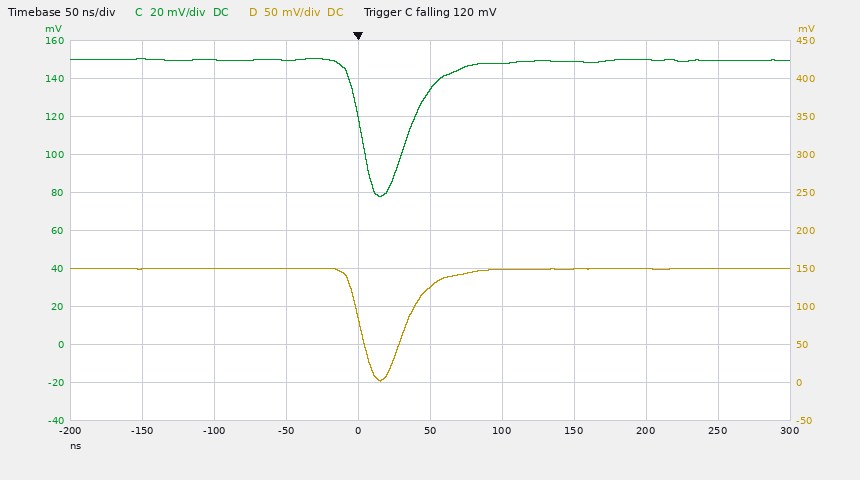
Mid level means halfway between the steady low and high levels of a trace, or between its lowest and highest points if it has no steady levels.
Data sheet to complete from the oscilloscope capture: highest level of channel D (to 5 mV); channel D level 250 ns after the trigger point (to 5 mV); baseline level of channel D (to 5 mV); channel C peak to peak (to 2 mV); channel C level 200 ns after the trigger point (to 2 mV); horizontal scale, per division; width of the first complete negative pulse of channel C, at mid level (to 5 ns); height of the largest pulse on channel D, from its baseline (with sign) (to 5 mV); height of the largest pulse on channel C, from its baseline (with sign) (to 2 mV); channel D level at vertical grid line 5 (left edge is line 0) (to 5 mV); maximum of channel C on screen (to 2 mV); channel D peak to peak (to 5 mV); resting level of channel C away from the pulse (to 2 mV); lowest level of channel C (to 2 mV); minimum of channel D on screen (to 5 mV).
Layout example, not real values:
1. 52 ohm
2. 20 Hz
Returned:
1. 150 mV
2. 150 mV
3. 150 mV
4. 72 mV
5. 150 mV
6. 50 ns
7. 35 ns
8. -150 mV
9. -72 mV
10. 125 mV
11. 150 mV
12. 150 mV
13. 150 mV
14. 78 mV
15. 0 mV
